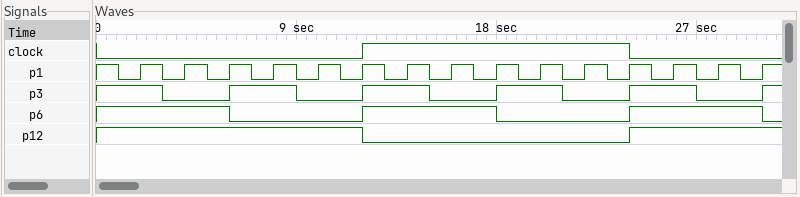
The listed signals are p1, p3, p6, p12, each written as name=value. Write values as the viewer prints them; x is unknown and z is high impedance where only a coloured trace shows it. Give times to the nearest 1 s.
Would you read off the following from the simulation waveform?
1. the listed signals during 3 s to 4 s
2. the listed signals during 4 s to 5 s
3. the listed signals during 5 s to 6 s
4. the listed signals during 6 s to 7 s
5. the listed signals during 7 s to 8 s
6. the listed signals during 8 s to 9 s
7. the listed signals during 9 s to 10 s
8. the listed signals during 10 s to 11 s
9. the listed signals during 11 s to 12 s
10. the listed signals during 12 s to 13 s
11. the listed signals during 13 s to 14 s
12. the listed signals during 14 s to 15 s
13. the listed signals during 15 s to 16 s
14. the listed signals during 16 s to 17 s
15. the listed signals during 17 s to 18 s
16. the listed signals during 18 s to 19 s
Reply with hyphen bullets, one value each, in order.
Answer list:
- p1=0, p3=0, p6=1, p12=1
- p1=1, p3=0, p6=1, p12=1
- p1=0, p3=0, p6=1, p12=1
- p1=1, p3=1, p6=0, p12=1
- p1=0, p3=1, p6=0, p12=1
- p1=1, p3=1, p6=0, p12=1
- p1=0, p3=0, p6=0, p12=1
- p1=1, p3=0, p6=0, p12=1
- p1=0, p3=0, p6=0, p12=1
- p1=1, p3=1, p6=1, p12=0
- p1=0, p3=1, p6=1, p12=0
- p1=1, p3=1, p6=1, p12=0
- p1=0, p3=0, p6=1, p12=0
- p1=1, p3=0, p6=1, p12=0
- p1=0, p3=0, p6=1, p12=0
- p1=1, p3=1, p6=0, p12=0
